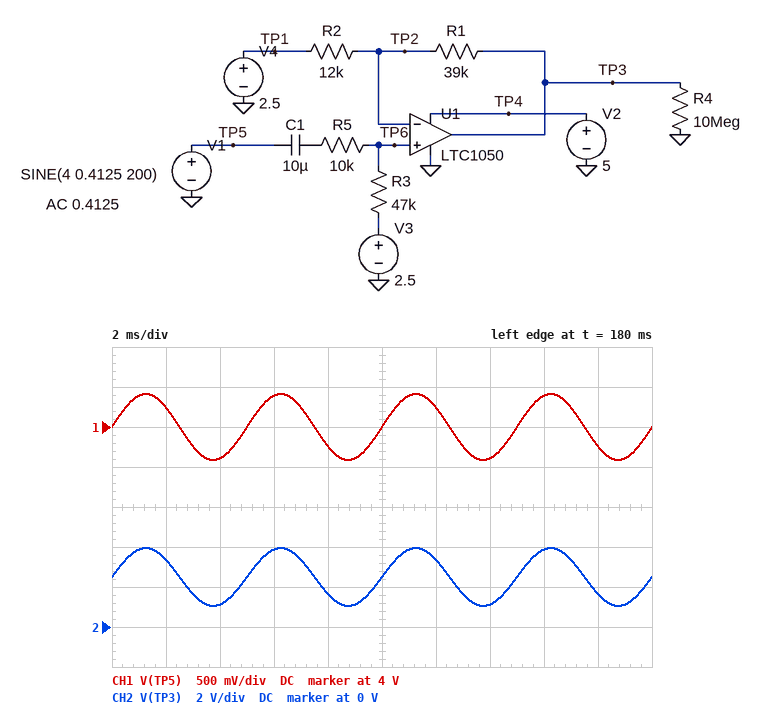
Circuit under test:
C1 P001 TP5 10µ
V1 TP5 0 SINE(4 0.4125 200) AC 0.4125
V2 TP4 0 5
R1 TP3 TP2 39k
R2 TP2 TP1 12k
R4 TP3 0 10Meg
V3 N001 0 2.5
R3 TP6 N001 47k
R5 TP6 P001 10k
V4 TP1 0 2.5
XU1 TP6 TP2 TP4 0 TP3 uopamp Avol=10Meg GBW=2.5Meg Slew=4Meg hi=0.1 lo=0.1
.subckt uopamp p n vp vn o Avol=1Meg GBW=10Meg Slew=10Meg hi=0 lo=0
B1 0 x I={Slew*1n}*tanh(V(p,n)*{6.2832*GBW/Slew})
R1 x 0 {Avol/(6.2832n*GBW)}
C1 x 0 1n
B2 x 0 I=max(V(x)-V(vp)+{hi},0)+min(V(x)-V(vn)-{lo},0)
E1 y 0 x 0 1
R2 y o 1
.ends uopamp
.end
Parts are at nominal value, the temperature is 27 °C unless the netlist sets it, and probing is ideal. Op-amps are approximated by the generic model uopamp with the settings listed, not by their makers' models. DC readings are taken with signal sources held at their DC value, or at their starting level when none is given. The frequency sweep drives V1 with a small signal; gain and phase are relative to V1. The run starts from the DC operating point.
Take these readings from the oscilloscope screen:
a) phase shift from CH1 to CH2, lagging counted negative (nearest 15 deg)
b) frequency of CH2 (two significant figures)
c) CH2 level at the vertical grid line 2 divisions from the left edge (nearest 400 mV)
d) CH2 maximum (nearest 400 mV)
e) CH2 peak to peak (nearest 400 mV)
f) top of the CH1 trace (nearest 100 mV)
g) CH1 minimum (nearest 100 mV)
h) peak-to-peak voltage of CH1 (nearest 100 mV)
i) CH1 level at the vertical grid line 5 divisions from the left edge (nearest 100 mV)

0 deg
200 Hz
1.2 V
4.0 V
2.8 V
4.4 V
3.6 V
800 mV
4.0 V
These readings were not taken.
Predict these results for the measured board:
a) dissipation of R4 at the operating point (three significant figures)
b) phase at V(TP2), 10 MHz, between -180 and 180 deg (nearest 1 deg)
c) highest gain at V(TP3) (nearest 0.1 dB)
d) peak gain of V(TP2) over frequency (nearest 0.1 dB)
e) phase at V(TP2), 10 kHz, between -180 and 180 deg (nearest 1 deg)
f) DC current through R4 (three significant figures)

625 nW
-87 deg
10.9 dB
-1.7 dB
-1 deg
250 nA
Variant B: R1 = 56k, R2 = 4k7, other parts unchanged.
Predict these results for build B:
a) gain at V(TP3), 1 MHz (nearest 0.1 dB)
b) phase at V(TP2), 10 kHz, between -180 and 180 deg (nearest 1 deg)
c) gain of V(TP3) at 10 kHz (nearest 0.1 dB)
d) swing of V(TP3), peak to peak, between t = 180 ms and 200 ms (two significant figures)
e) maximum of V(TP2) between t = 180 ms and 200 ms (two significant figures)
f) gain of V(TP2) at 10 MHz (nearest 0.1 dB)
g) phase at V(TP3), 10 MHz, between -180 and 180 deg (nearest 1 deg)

6.1 dB
-3 deg
20.5 dB
4.8 V
2.7 V
-35.9 dB
-89 deg
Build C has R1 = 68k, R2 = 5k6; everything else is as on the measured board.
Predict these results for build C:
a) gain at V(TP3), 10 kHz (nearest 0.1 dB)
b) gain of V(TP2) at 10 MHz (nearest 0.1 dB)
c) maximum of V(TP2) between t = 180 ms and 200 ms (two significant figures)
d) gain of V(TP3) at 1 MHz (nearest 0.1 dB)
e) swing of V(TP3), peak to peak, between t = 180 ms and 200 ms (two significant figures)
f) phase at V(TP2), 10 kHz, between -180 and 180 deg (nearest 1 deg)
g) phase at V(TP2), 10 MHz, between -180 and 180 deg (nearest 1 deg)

20.7 dB
-36.1 dB
2.7 V
6.1 dB
4.8 V
-3 deg
-89 deg
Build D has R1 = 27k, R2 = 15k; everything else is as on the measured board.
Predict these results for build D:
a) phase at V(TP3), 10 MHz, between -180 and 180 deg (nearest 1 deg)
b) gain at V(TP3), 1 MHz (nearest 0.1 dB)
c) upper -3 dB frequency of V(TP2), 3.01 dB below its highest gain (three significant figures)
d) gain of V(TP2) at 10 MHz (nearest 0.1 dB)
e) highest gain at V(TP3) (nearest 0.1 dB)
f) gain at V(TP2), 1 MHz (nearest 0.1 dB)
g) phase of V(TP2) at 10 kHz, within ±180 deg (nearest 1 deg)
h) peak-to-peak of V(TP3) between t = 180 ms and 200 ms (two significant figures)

-85 deg
3.7 dB
893 kHz
-22.7 dB
7.3 dB
-5.2 dB
-1 deg
1.9 V
